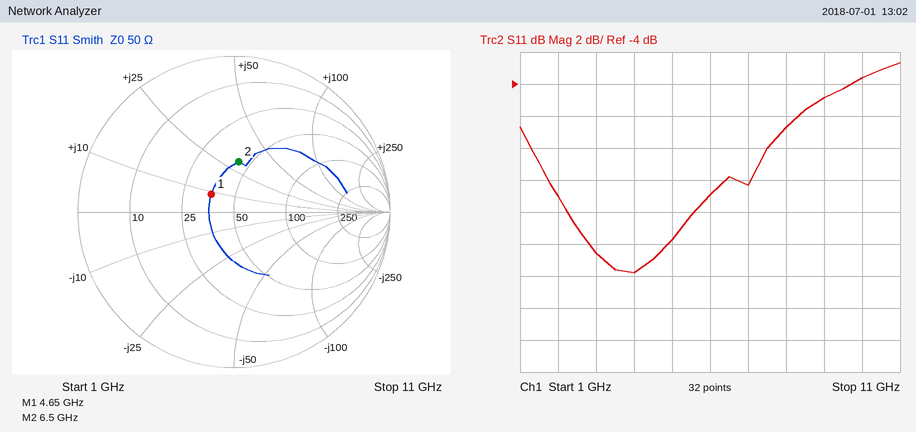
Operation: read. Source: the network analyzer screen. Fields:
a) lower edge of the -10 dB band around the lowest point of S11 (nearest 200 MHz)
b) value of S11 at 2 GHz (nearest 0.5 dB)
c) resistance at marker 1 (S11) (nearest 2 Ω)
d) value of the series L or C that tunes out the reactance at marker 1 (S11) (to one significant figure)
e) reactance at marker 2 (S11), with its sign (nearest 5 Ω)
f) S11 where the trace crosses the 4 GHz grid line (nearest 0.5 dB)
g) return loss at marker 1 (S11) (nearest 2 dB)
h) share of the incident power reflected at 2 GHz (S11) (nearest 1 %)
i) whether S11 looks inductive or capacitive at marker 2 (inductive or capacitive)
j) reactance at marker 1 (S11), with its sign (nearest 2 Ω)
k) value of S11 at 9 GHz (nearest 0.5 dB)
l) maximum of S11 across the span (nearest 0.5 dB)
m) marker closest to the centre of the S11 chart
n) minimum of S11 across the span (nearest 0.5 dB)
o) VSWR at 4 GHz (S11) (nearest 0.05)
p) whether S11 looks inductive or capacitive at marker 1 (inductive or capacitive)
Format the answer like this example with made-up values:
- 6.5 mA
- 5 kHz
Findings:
- 1.8 GHz
- -11.0 dB
- 36 Ω
- 4 pF
- +30 Ω
- -16.0 dB
- 14 dB
- 8 %
- inductive
- +8 Ω
- -5.0 dB
- -2.5 dB
- marker 1
- -16.0 dB
- 1.40
- inductive
